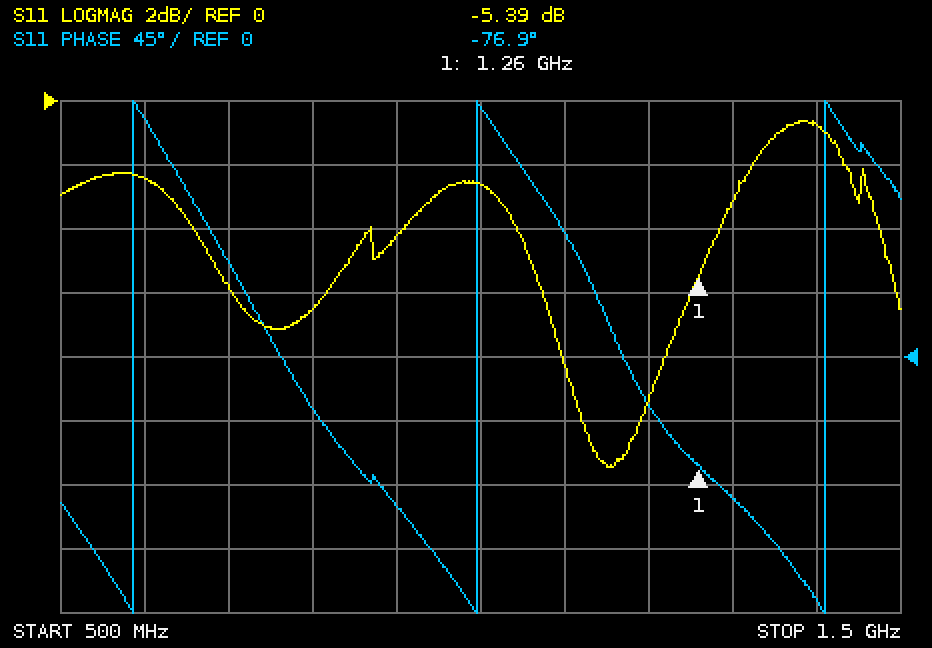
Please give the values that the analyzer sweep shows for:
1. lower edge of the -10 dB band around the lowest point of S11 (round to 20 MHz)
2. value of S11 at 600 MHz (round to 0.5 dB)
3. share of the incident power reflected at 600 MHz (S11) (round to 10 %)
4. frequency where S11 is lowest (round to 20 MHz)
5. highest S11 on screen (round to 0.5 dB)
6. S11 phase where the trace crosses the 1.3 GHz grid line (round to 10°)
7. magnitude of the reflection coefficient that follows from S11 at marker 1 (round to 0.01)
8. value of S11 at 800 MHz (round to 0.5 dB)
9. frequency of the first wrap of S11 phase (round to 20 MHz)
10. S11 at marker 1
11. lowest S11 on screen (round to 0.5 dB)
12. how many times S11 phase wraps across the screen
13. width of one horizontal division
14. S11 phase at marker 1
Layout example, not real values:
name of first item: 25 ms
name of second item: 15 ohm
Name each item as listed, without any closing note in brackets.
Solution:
lower edge of the -10 dB band around the lowest point of S11: 1.12 GHz
value of S11 at 600 MHz: -2.5 dB
share of the incident power reflected at 600 MHz (S11): 60 %
frequency where S11 is lowest: 1.16 GHz
highest S11 on screen: -0.5 dB
S11 phase where the trace crosses the 1.3 GHz grid line: -100°
magnitude of the reflection coefficient that follows from S11 at marker 1: 0.54
value of S11 at 800 MHz: -6.5 dB
frequency of the first wrap of S11 phase: 580 MHz
S11 at marker 1: -5.39 dB
lowest S11 on screen: -11.5 dB
how many times S11 phase wraps across the screen: 3
width of one horizontal division: 100 MHz
S11 phase at marker 1: -76.9°
